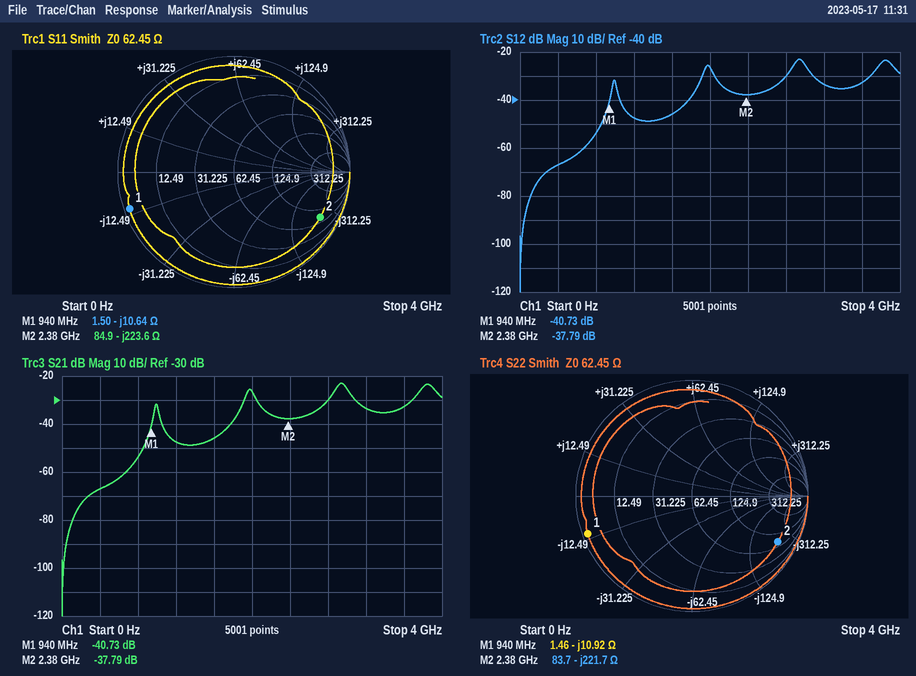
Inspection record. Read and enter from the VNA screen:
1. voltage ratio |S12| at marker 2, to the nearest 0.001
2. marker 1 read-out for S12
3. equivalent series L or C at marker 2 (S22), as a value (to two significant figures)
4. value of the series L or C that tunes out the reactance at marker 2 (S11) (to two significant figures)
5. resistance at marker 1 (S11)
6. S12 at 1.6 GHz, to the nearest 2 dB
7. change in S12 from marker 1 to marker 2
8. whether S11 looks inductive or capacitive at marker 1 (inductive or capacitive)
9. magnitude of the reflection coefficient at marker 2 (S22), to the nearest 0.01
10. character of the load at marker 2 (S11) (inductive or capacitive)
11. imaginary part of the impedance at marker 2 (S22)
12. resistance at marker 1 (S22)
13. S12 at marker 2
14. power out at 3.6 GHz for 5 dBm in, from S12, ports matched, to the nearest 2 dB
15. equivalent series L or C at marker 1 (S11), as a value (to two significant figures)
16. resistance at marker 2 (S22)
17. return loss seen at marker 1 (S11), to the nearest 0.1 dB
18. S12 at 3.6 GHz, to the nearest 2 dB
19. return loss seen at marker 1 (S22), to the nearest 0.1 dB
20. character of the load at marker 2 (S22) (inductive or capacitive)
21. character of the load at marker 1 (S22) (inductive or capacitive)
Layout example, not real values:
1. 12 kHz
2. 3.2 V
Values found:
1. 0.013
2. -40.73 dB
3. 300 fF
4. 15 nH
5. 1.50 Ω
6. -46 dB
7. 2.94 dB
8. capacitive
9. 0.84
10. capacitive
11. -221.7 Ω
12. 1.46 Ω
13. -37.79 dB
14. -28 dBm
15. 16 pF
16. 83.7 Ω
17. 0.4 dB
18. -32 dB
19. 0.4 dB
20. capacitive
21. capacitive
